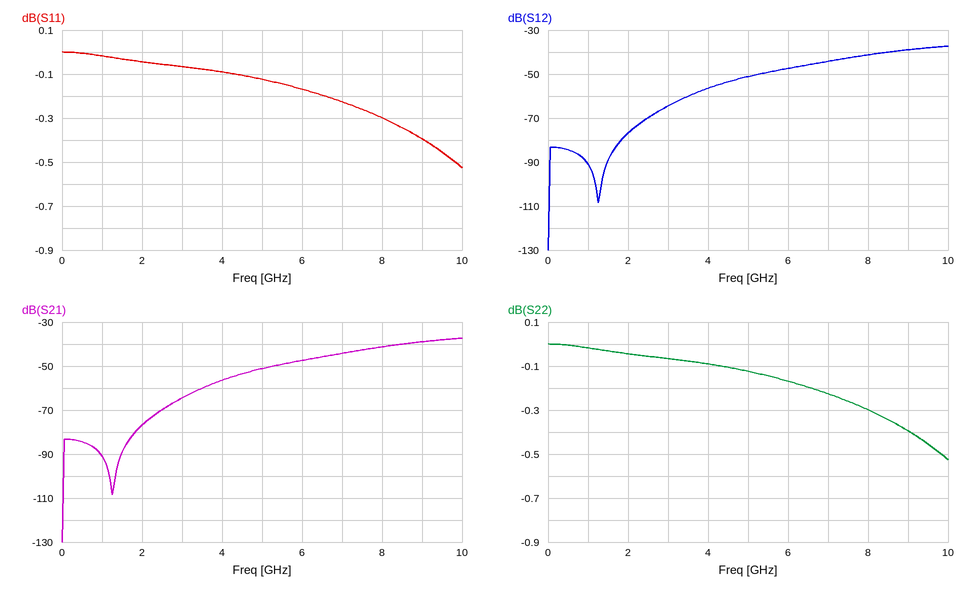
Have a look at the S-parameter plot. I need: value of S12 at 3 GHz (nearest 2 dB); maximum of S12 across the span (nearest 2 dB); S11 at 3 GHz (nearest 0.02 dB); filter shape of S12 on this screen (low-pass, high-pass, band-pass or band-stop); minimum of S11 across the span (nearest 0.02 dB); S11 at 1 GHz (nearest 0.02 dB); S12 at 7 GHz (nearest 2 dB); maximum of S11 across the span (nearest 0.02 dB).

-64 dB
-38 dB
-0.06 dB
high-pass
-0.52 dB
-0.02 dB
-44 dB
0.00 dB
